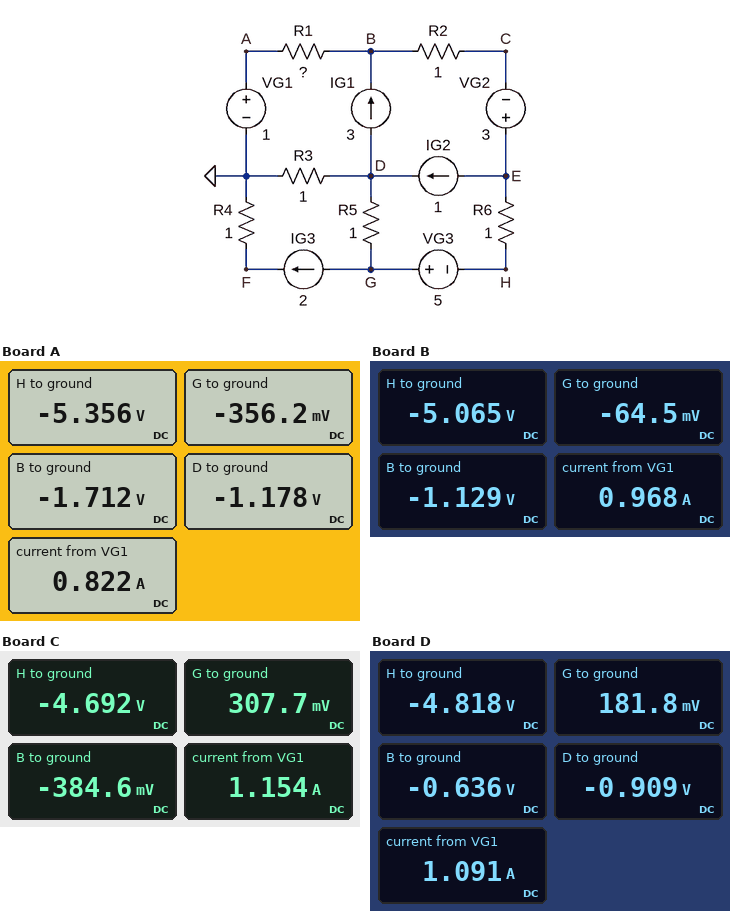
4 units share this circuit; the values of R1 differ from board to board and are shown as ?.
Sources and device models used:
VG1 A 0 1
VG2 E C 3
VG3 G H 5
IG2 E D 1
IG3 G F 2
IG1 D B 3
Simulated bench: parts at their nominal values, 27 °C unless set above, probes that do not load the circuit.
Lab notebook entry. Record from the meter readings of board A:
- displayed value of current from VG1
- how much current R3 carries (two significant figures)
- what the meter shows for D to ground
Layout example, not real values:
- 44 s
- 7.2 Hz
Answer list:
- 0.822 A
- 1.2 A
- -1.178 V
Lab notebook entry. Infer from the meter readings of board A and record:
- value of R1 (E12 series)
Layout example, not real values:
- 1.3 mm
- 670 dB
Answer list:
- 3.3 Ω
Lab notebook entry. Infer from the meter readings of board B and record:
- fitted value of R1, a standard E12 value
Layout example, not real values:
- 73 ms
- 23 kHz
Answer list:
- 2.2 Ω
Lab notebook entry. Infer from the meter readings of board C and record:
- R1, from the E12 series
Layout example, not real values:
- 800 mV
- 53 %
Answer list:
- 1.2 Ω
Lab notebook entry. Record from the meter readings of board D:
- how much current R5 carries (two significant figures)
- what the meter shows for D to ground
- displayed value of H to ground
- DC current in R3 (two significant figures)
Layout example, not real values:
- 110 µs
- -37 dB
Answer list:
- 1.1 A
- -0.909 V
- -4.818 V
- 910 mA
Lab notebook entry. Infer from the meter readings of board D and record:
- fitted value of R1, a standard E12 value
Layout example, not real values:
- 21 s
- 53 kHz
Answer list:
- 1.5 Ω
